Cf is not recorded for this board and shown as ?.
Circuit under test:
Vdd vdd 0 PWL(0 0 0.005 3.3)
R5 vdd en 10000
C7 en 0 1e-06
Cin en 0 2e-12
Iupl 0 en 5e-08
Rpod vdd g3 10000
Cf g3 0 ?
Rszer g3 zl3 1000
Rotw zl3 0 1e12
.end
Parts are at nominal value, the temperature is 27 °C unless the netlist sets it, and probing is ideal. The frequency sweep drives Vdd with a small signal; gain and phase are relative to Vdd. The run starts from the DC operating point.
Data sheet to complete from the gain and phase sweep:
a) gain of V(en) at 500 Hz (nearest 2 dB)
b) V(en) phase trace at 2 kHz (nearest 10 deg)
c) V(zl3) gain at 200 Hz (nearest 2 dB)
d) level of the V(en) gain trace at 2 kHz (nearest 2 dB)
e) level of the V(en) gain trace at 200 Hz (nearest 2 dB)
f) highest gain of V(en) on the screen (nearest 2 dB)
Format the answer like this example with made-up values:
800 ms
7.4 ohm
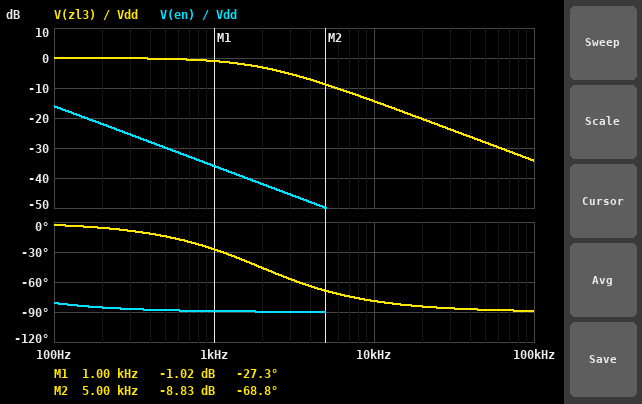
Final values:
-30 dB
-90 deg
0 dB
-42 dB
-22 dB
-16 dB
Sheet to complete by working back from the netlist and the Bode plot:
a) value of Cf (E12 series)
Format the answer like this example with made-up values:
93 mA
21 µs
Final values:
8.2 nF
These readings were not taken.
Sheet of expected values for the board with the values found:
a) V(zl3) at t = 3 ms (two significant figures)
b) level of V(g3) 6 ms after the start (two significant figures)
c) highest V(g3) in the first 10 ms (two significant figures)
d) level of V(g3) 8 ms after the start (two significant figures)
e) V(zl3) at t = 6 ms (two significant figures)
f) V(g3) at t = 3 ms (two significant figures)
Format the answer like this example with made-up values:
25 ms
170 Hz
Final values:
1.9 V
3.3 V
3.3 V
3.3 V
3.3 V
1.9 V
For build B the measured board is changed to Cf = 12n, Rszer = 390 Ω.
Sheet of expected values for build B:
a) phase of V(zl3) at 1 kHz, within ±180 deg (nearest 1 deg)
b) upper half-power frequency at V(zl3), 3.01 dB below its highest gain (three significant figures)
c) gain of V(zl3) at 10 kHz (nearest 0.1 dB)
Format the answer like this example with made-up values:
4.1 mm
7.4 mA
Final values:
-37 deg
1.33 kHz
-17.6 dB
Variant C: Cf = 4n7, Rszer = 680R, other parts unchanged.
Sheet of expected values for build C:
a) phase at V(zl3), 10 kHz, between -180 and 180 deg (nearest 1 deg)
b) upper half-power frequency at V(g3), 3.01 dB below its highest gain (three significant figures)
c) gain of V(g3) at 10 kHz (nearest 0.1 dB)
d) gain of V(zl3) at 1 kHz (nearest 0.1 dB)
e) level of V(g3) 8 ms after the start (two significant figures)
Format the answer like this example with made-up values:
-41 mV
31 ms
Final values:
-71 deg
3.39 kHz
-9.9 dB
-0.4 dB
3.3 V
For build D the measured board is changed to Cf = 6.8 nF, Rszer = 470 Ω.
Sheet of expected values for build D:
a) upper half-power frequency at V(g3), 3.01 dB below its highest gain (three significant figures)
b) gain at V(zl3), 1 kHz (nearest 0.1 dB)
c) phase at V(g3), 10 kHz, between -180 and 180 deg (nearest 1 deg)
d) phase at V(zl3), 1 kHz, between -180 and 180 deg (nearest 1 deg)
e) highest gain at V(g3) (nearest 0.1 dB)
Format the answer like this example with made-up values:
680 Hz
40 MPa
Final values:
2.34 kHz
-0.7 dB
-77 deg
-23 deg
0 dB
